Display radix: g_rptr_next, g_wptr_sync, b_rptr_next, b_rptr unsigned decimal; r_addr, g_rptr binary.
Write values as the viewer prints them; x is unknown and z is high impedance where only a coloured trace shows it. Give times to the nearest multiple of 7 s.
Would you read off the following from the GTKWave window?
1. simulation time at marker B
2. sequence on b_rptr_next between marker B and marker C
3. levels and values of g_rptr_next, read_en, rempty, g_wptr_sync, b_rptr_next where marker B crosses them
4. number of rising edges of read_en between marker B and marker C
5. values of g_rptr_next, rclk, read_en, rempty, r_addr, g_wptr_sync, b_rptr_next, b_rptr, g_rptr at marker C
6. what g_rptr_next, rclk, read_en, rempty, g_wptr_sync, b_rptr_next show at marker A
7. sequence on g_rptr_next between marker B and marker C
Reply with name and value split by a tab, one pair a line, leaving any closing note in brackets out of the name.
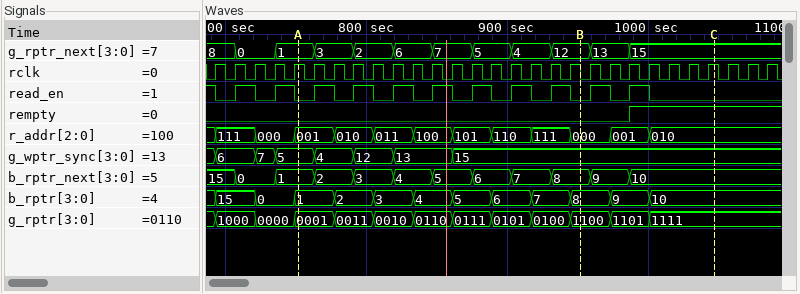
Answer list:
simulation time at marker B	952 s
sequence on b_rptr_next between marker B and marker C	8, 9, 10
levels and values of g_rptr_next, read_en, rempty, g_wptr_sync, b_rptr_next where marker B crosses them	g_rptr_next=12, read_en=0, rempty=0, g_wptr_sync=15, b_rptr_next=8
number of rising edges of read_en between marker B and marker C	2
values of g_rptr_next, rclk, read_en, rempty, r_addr, g_wptr_sync, b_rptr_next, b_rptr, g_rptr at marker C	g_rptr_next=15, rclk=1, read_en=0, rempty=1, r_addr=010, g_wptr_sync=15, b_rptr_next=10, b_rptr=10, g_rptr=1111
what g_rptr_next, rclk, read_en, rempty, g_wptr_sync, b_rptr_next show at marker A	g_rptr_next=1, rclk=1, read_en=0, rempty=0, g_wptr_sync=5, b_rptr_next=1
sequence on g_rptr_next between marker B and marker C	12, 13, 15
